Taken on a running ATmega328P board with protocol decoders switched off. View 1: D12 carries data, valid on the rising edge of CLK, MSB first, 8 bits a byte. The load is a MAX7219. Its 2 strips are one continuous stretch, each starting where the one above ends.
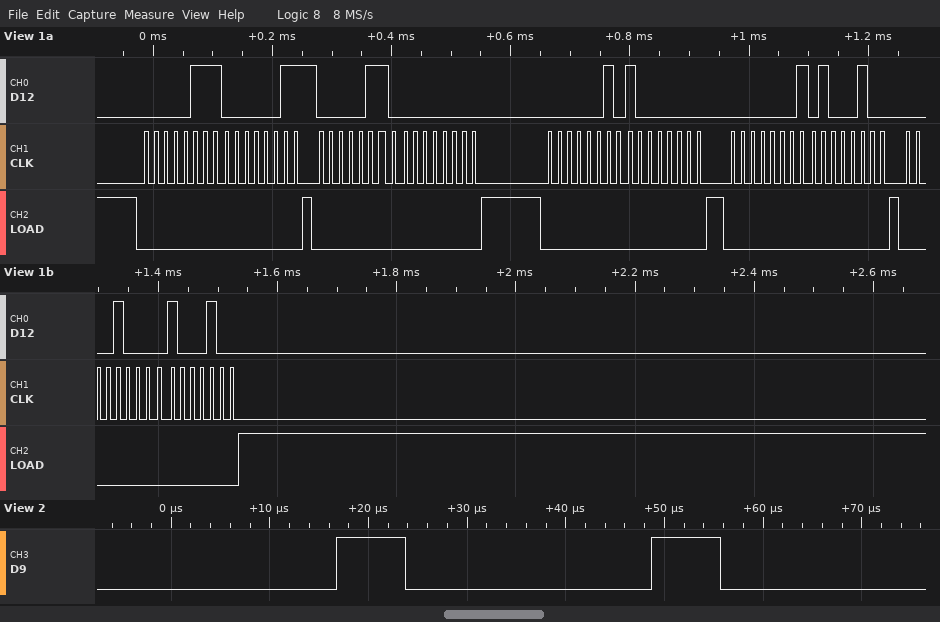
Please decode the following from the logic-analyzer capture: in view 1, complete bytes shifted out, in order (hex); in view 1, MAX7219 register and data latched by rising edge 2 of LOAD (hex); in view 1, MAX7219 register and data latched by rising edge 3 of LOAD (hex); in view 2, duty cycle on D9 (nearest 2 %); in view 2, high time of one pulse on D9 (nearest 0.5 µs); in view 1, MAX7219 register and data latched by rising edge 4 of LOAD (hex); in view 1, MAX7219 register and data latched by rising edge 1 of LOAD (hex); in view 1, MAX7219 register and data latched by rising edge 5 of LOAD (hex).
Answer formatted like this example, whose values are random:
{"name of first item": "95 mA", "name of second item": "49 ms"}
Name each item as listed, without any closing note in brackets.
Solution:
{"in view 1, complete bytes shifted out, in order": "07 03 06 00 02 80 01 44 08 44", "in view 1, MAX7219 register and data latched by rising edge 2 of LOAD": "register 0x6, data 0x00", "in view 1, MAX7219 register and data latched by rising edge 3 of LOAD": "register 0x2, data 0x80", "in view 2, duty cycle on D9": "22 %", "in view 2, high time of one pulse on D9": "7.0 µs", "in view 1, MAX7219 register and data latched by rising edge 4 of LOAD": "register 0x1, data 0x44", "in view 1, MAX7219 register and data latched by rising edge 1 of LOAD": "register 0x7, data 0x03", "in view 1, MAX7219 register and data latched by rising edge 5 of LOAD": "register 0x8, data 0x44"}
